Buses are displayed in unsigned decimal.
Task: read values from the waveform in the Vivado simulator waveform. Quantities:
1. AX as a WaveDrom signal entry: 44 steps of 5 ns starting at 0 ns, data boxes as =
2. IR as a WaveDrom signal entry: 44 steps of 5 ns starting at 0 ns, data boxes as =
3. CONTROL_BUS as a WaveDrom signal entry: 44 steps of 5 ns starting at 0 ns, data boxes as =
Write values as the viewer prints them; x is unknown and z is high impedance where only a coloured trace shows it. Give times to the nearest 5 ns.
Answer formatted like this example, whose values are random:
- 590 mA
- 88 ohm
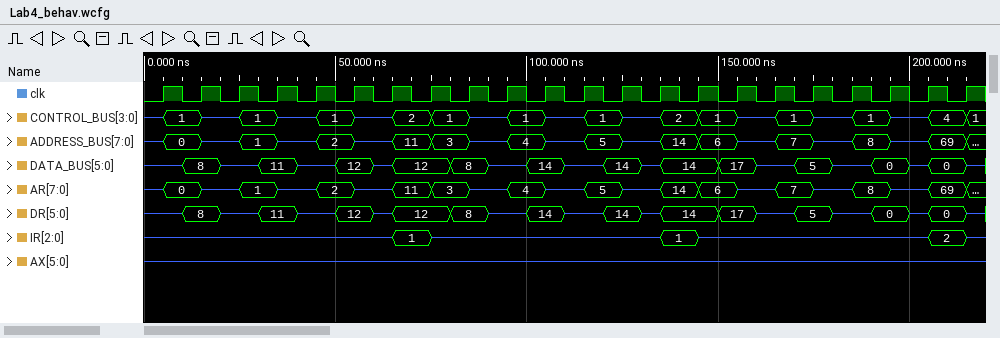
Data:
- {name: 'AX', wave: 'z...........................................'}
- {name: 'IR', wave: 'z............=.z...........=.z...........=.z', data: '1 1 2'}
- {name: 'CONTROL_BUS', wave: 'z=.z.=.z.=.z.=.=.z.=.z.=.z.=.=.z.=.z.=.z.=.=', data: '1 1 1 2 1 1 1 2 1 1 1 4 1'}
